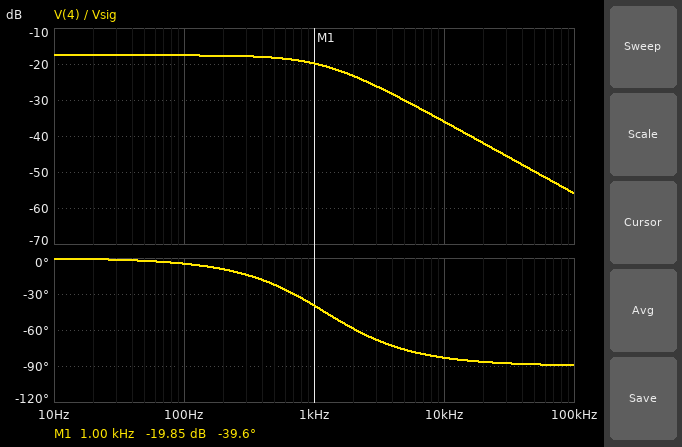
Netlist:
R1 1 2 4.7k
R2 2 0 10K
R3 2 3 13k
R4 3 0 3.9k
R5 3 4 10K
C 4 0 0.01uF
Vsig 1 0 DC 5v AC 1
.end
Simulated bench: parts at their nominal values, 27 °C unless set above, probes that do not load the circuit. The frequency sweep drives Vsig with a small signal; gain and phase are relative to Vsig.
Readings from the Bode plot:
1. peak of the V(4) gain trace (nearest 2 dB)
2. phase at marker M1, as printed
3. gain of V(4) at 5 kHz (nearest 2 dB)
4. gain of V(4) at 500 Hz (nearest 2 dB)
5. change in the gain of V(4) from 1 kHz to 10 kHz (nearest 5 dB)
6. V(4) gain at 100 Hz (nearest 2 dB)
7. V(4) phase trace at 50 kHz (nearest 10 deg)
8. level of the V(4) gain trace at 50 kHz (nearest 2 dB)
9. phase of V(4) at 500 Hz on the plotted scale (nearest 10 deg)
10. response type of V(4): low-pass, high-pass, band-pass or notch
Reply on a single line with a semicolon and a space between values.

-18 dB; -39.6 deg; -30 dB; -18 dB; -15 dB; -18 dB; -90 deg; -50 dB; -20 deg; low-pass
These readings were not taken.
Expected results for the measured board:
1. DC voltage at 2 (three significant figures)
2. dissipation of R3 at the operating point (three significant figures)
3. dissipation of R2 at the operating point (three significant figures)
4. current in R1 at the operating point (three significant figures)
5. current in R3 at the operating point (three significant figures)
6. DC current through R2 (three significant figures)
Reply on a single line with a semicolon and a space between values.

2.86 V; 372 µW; 818 µW; 455 µA; 169 µA; 286 µA
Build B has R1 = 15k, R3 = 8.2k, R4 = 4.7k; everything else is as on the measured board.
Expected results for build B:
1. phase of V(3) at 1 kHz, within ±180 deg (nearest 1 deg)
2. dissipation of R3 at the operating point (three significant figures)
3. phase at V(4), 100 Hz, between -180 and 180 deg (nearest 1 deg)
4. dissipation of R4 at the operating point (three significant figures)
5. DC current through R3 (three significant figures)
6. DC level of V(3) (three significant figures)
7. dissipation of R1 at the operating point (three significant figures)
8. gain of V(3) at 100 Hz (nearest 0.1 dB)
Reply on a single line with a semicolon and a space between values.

-8 deg; 91.8 µW; -5 deg; 52.6 µW; 106 µA; 497 mV; 881 µW; -20.1 dB
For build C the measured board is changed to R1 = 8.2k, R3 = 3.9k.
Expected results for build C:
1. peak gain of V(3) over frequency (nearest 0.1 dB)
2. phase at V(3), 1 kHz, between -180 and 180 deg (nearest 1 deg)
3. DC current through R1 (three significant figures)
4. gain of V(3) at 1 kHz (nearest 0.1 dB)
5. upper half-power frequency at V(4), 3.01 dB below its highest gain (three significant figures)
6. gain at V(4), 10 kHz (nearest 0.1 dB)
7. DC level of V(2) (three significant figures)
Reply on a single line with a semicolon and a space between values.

-15.2 dB; -6 deg; 397 µA; -15.9 dB; 1.26 kHz; -33.3 dB; 1.74 V
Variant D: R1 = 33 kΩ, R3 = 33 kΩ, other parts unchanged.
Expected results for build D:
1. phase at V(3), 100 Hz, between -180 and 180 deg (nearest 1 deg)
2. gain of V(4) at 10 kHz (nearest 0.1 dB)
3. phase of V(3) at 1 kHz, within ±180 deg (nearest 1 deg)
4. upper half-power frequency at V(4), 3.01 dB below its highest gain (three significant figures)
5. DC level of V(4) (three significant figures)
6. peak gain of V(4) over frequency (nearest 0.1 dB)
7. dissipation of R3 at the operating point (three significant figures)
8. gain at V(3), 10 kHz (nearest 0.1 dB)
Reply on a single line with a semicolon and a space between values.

-1 deg; -52.5 dB; -8 deg; 1.17 kHz; 102 mV; -33.8 dB; 22.5 µW; -36.4 dB
